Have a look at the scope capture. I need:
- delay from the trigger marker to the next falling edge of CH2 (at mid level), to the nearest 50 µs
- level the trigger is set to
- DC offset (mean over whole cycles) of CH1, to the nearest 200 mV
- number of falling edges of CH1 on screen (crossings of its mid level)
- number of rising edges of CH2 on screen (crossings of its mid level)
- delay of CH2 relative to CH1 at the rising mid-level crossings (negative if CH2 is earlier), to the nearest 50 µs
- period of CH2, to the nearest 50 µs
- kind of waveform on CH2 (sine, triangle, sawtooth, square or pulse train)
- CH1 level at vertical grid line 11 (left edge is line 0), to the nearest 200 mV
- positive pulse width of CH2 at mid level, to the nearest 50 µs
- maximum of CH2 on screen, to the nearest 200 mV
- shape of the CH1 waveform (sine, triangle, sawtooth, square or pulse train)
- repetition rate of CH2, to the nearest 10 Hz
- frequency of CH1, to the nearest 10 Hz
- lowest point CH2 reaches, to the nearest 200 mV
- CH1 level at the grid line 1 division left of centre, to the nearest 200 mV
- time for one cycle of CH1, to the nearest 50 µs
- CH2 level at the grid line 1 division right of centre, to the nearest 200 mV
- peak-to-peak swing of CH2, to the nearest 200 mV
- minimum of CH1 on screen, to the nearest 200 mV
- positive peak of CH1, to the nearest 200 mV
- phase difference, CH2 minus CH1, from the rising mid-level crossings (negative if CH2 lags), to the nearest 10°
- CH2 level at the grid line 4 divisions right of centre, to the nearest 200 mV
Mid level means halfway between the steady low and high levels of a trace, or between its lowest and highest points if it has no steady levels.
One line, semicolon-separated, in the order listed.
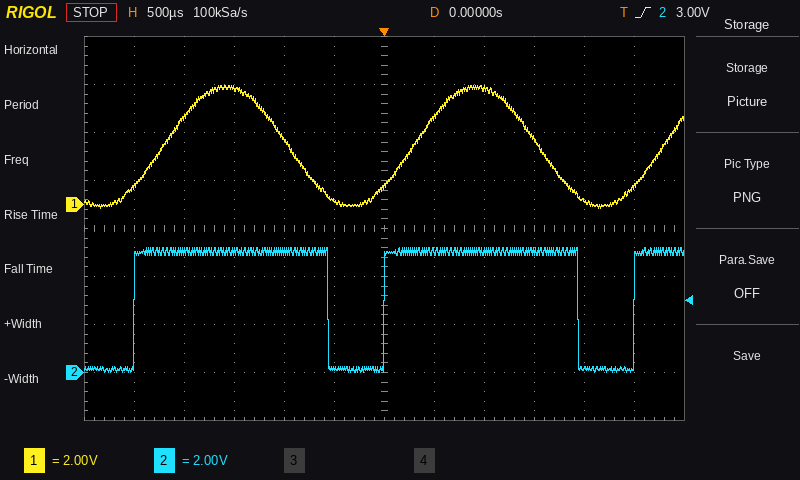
1.95 ms; 3.00 V; 2.4 V; 2; 3; -300 µs; 2.50 ms; pulse train; 800 mV; 1.95 ms; 5.2 V; sine; 400 Hz; 400 Hz; 0.0 V; 200 mV; 2.50 ms; 5.0 V; 5.2 V; -200 mV; 5.0 V; +40°; 200 mV
